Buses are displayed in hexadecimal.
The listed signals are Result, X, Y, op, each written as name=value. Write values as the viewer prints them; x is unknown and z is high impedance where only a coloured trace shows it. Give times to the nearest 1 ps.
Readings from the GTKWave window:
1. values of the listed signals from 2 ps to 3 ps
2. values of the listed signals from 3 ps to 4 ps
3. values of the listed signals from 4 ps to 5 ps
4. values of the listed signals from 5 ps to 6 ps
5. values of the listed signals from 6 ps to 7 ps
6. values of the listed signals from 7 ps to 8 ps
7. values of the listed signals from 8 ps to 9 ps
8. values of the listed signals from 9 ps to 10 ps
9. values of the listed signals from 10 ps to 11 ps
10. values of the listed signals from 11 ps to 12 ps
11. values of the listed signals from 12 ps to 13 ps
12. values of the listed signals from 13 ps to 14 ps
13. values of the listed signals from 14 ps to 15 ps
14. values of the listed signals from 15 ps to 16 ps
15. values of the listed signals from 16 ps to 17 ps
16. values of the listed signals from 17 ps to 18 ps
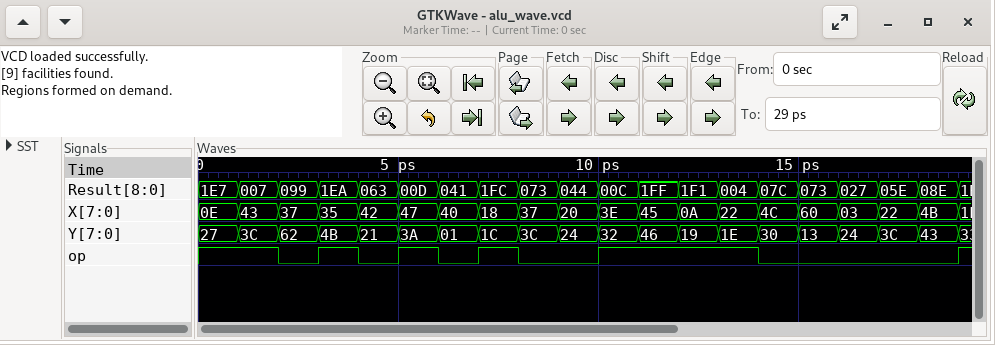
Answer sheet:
Result=099, X=37, Y=62, op=0
Result=1EA, X=35, Y=4B, op=1
Result=063, X=42, Y=21, op=0
Result=00D, X=47, Y=3A, op=1
Result=041, X=40, Y=01, op=0
Result=1FC, X=18, Y=1C, op=1
Result=073, X=37, Y=3C, op=0
Result=044, X=20, Y=24, op=0
Result=00C, X=3E, Y=32, op=1
Result=1FF, X=45, Y=46, op=1
Result=1F1, X=0A, Y=19, op=1
Result=004, X=22, Y=1E, op=1
Result=07C, X=4C, Y=30, op=0
Result=073, X=60, Y=13, op=0
Result=027, X=03, Y=24, op=0
Result=05E, X=22, Y=3C, op=0
